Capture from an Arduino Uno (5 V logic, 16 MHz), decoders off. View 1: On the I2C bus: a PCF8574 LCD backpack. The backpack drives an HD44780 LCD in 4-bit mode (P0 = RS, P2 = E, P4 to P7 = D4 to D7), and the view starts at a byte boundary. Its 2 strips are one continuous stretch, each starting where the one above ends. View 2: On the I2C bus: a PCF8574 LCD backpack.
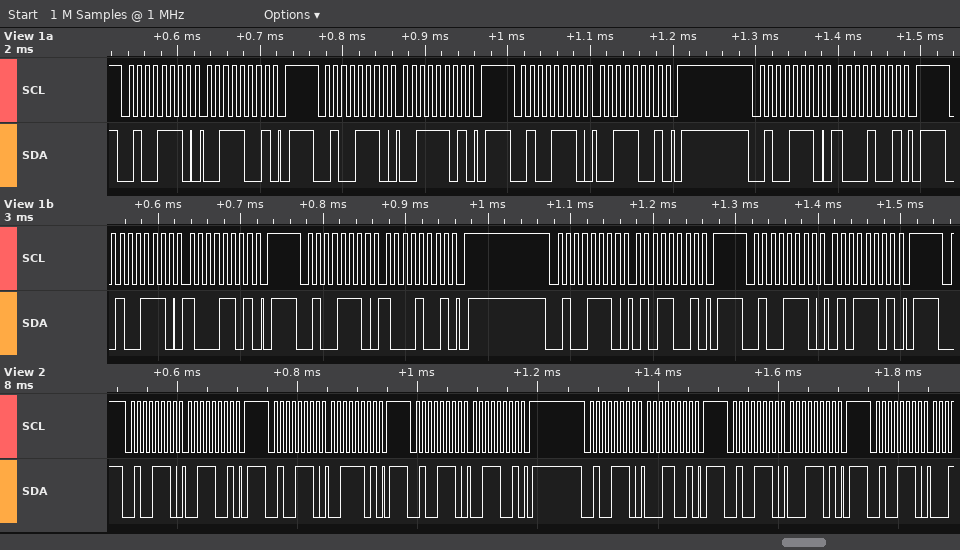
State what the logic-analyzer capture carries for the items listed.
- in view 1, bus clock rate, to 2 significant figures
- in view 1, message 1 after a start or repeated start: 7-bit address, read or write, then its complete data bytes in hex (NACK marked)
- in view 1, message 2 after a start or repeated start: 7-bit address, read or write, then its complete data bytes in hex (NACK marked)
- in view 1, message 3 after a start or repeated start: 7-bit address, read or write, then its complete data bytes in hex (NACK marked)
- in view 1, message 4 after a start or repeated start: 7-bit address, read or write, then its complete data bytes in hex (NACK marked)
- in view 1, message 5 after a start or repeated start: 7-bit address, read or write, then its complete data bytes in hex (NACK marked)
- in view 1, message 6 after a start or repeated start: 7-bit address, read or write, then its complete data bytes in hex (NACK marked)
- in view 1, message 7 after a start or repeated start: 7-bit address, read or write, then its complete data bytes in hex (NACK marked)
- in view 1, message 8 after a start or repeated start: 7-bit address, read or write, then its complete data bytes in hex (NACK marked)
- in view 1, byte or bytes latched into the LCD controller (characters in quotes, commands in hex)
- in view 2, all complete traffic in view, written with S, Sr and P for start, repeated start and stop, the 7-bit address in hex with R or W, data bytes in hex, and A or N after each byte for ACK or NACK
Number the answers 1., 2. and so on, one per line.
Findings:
1. 100 kHz
2. 0x27 write: 39
3. 0x27 write: 3D
4. 0x27 write: 39
5. 0x27 write: 89
6. 0x27 write: 8D
7. 0x27 write: 89
8. 0x27 write: 59
9. 0x27 write: 5D
10. '8'
11. S 27W A 39 A P S 27W A 3D A P S 27W A 39 A P S 27W A 19 A P S 27W A 1D A P S 27W A
